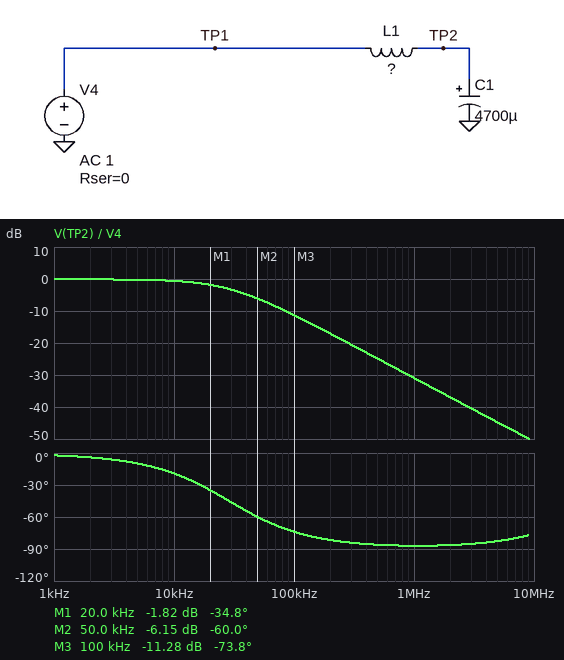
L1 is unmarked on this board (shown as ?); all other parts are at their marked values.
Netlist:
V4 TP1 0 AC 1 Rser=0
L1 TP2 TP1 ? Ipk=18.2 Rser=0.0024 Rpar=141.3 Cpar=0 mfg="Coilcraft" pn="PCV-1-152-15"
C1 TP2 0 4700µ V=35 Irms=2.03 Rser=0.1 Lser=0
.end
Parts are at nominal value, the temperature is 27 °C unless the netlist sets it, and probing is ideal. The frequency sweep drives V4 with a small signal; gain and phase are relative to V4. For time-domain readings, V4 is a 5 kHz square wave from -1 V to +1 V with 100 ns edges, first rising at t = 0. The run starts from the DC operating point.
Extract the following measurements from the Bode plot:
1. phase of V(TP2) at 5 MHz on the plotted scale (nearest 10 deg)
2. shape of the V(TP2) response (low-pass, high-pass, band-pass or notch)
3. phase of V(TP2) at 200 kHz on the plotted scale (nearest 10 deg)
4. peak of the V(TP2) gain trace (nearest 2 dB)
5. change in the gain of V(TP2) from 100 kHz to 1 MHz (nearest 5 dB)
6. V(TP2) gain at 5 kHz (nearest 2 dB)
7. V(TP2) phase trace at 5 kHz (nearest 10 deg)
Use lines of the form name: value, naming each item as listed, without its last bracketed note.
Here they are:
phase of V(TP2) at 5 MHz on the plotted scale: -80 deg
shape of the V(TP2) response: low-pass
phase of V(TP2) at 200 kHz on the plotted scale: -80 deg
peak of the V(TP2) gain trace: 0 dB
change in the gain of V(TP2) from 100 kHz to 1 MHz: -20 dB
V(TP2) gain at 5 kHz: 0 dB
V(TP2) phase trace at 5 kHz: -10 deg
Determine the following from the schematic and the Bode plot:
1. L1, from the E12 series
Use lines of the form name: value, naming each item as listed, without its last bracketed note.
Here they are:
L1, from the E12 series: 560 nH
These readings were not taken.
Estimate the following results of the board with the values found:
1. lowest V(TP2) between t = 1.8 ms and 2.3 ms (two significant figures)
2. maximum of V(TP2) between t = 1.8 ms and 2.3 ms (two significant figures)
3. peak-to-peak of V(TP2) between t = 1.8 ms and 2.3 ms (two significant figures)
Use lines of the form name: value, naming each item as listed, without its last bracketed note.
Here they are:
lowest V(TP2) between t = 1.8 ms and 2.3 ms: -990 mV
maximum of V(TP2) between t = 1.8 ms and 2.3 ms: 990 mV
peak-to-peak of V(TP2) between t = 1.8 ms and 2.3 ms: 2.0 V
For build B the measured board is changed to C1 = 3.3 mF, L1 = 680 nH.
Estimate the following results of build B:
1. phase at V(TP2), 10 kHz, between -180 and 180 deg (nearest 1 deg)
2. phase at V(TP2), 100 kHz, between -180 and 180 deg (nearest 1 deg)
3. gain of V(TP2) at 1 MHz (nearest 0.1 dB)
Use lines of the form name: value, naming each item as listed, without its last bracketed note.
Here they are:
phase at V(TP2), 10 kHz, between -180 and 180 deg: -23 deg
phase at V(TP2), 100 kHz, between -180 and 180 deg: -77 deg
gain of V(TP2) at 1 MHz: -32.6 dB
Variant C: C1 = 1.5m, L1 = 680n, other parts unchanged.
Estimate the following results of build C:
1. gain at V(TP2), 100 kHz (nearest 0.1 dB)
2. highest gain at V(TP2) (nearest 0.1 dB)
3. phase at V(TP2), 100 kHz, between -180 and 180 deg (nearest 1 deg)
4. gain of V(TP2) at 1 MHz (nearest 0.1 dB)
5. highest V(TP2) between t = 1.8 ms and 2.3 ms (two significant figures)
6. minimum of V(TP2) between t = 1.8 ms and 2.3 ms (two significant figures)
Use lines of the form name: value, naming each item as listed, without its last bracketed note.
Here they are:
gain at V(TP2), 100 kHz: -12.8 dB
highest gain at V(TP2): 0.1 dB
phase at V(TP2), 100 kHz, between -180 and 180 deg: -77 deg
gain of V(TP2) at 1 MHz: -32.6 dB
highest V(TP2) between t = 1.8 ms and 2.3 ms: 1.0 V
minimum of V(TP2) between t = 1.8 ms and 2.3 ms: -1.0 V
